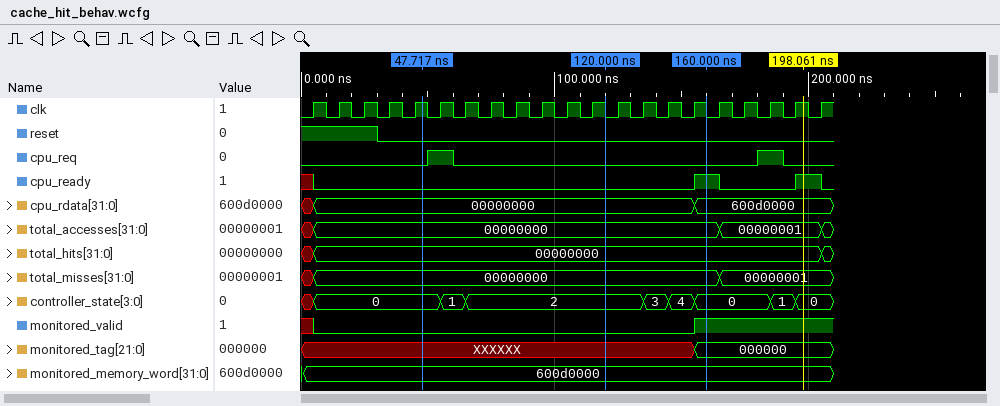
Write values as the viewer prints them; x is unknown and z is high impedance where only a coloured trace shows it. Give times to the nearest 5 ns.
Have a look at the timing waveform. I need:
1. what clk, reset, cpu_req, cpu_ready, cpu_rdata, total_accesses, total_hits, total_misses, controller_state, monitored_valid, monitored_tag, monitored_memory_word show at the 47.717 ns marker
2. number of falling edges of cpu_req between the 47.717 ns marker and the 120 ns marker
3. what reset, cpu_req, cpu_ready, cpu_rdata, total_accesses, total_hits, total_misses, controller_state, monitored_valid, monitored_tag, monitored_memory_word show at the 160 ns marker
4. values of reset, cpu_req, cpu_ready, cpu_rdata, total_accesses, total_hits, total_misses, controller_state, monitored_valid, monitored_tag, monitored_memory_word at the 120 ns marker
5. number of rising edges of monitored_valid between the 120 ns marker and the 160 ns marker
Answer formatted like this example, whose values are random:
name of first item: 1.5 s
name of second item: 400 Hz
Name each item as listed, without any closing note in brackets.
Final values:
what clk, reset, cpu_req, cpu_ready, cpu_rdata, total_accesses, total_hits, total_misses, controller_state, monitored_valid, monitored_tag, monitored_memory_word show at the 47.717 ns marker: clk=1, reset=0, cpu_req=0, cpu_ready=0, cpu_rdata=00000000, total_accesses=00000000, total_hits=00000000, total_misses=00000000, controller_state=0, monitored_valid=0, monitored_tag=XXXXXX, monitored_memory_word=600d0000
number of falling edges of cpu_req between the 47.717 ns marker and the 120 ns marker: 1
what reset, cpu_req, cpu_ready, cpu_rdata, total_accesses, total_hits, total_misses, controller_state, monitored_valid, monitored_tag, monitored_memory_word show at the 160 ns marker: reset=0, cpu_req=0, cpu_ready=1, cpu_rdata=600d0000, total_accesses=00000000, total_hits=00000000, total_misses=00000000, controller_state=0, monitored_valid=1, monitored_tag=000000, monitored_memory_word=600d0000
values of reset, cpu_req, cpu_ready, cpu_rdata, total_accesses, total_hits, total_misses, controller_state, monitored_valid, monitored_tag, monitored_memory_word at the 120 ns marker: reset=0, cpu_req=0, cpu_ready=0, cpu_rdata=00000000, total_accesses=00000000, total_hits=00000000, total_misses=00000000, controller_state=2, monitored_valid=0, monitored_tag=XXXXXX, monitored_memory_word=600d0000
number of rising edges of monitored_valid between the 120 ns marker and the 160 ns marker: 1
